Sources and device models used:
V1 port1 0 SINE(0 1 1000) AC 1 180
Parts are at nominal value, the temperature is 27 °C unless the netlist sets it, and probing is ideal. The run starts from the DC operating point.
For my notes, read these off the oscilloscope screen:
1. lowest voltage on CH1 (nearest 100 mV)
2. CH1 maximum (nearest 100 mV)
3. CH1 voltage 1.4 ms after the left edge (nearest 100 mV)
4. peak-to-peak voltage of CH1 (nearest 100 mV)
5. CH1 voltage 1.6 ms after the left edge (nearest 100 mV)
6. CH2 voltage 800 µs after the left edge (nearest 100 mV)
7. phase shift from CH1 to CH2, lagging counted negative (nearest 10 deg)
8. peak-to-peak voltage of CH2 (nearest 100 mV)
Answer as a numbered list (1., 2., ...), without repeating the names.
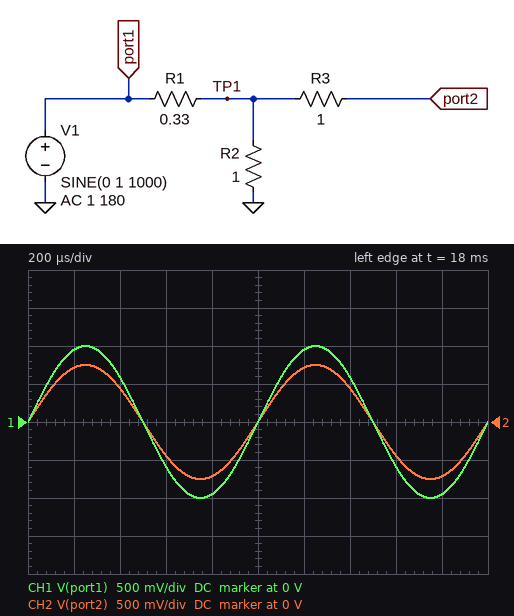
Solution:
1. -1.0 V
2. 1.0 V
3. 600 mV
4. 2.0 V
5. -600 mV
6. -700 mV
7. 0 deg
8. 1.5 V
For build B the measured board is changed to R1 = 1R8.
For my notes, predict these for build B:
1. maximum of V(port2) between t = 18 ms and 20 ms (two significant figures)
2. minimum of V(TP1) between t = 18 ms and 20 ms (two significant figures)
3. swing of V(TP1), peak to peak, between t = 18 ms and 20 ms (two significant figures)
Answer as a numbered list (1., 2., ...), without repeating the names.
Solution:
1. 360 mV
2. -360 mV
3. 710 mV
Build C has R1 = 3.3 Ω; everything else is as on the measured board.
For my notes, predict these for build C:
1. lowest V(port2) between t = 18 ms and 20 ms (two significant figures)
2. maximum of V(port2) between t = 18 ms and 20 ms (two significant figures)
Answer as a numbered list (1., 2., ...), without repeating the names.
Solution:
1. -230 mV
2. 230 mV
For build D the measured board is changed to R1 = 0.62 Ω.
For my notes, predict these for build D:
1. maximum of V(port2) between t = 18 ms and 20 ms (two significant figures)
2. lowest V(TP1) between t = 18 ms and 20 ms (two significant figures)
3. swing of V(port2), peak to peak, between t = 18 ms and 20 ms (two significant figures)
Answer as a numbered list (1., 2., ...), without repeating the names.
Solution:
1. 620 mV
2. -620 mV
3. 1.2 V
